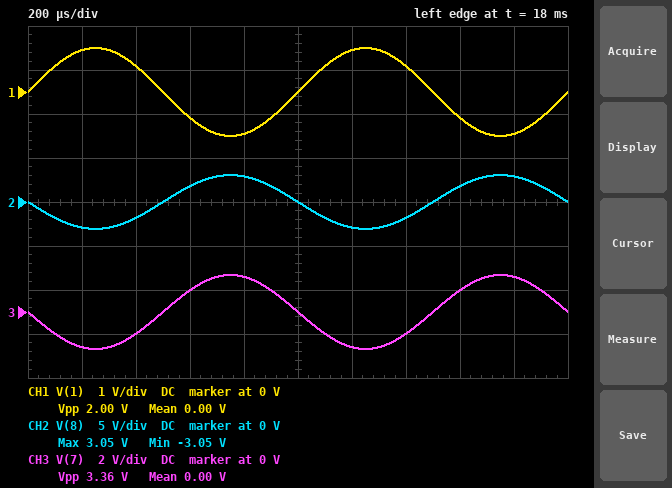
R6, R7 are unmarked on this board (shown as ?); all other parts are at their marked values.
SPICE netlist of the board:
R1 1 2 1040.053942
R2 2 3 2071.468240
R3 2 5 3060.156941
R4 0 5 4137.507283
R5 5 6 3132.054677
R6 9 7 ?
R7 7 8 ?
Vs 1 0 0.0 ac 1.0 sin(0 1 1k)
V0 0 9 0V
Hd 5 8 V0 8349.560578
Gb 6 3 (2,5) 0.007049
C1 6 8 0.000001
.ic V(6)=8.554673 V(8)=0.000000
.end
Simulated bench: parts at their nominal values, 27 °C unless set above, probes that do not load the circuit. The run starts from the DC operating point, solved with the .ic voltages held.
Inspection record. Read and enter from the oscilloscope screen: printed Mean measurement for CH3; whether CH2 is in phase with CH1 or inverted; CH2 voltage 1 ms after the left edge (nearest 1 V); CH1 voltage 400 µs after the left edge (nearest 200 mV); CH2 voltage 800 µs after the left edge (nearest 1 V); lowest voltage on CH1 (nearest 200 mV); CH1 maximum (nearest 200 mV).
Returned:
0.00 V
inverted
0 V
600 mV
3 V
-1.0 V
1.0 V
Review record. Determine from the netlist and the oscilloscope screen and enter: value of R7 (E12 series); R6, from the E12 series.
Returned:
2.7 kΩ
3.3 kΩ
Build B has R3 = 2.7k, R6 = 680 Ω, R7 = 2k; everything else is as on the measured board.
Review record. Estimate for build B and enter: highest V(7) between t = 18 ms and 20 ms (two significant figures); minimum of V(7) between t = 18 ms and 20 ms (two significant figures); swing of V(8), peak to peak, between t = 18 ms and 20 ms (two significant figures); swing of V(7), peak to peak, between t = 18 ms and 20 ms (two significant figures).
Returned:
110 mV
-110 mV
890 mV
230 mV
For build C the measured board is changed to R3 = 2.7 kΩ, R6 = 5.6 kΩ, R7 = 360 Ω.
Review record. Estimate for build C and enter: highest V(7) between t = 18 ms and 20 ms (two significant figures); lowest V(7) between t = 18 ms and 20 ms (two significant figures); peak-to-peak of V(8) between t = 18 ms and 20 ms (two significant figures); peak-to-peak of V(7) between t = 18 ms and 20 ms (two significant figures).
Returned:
2.8 V
-2.8 V
5.9 V
5.6 V
